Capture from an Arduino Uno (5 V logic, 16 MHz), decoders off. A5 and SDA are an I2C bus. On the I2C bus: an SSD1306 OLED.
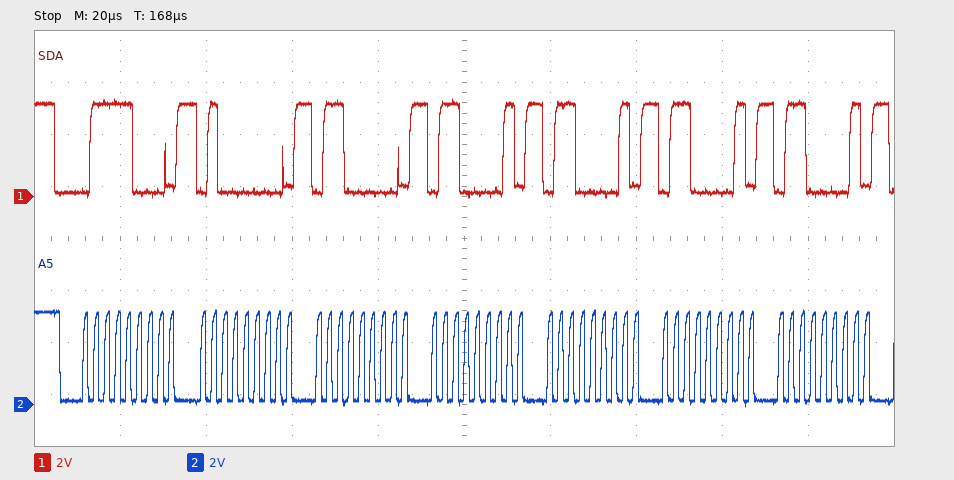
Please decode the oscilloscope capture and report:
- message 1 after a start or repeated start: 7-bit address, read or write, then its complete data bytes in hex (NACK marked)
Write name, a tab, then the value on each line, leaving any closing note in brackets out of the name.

message 1 after a start or repeated start: 7-bit address, read or write, then its complete data bytes in hex	0x3C write: 40 60 61 61 61 61
